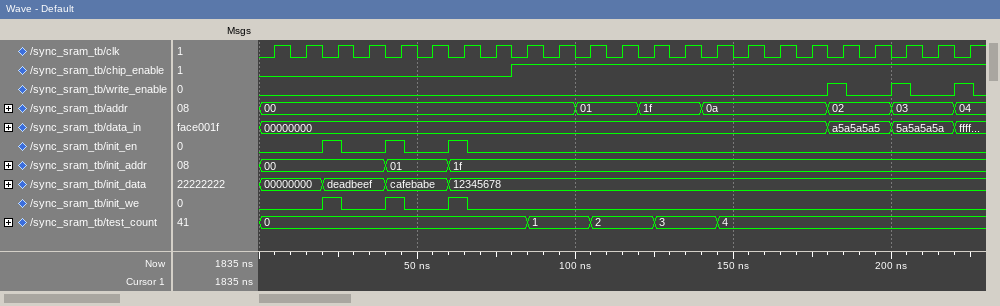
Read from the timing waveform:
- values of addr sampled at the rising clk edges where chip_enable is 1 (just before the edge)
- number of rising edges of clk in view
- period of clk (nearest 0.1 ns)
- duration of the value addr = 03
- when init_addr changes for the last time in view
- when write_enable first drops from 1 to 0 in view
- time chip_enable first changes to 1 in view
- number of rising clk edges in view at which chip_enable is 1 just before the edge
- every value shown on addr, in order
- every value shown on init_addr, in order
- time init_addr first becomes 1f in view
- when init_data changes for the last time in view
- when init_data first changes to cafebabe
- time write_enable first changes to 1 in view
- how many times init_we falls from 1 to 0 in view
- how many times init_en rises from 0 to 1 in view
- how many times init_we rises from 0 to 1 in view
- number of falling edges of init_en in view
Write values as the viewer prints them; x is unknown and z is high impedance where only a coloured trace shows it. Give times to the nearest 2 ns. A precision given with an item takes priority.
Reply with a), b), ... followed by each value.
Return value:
a) 00, 00, 01, 01, 1f, 1f, 0a, 0a, 0a, 0a, 02, 02, 03, 03, 04
b) 23
c) 10 ns
d) 20 ns
e) 60 ns
f) 186 ns
g) 80 ns
h) 15
i) 00, 01, 1f, 0a, 02, 03, 04
j) 00, 01, 1f
k) 60 ns
l) 60 ns
m) 40 ns
n) 180 ns
o) 3
p) 3
q) 3
r) 3
